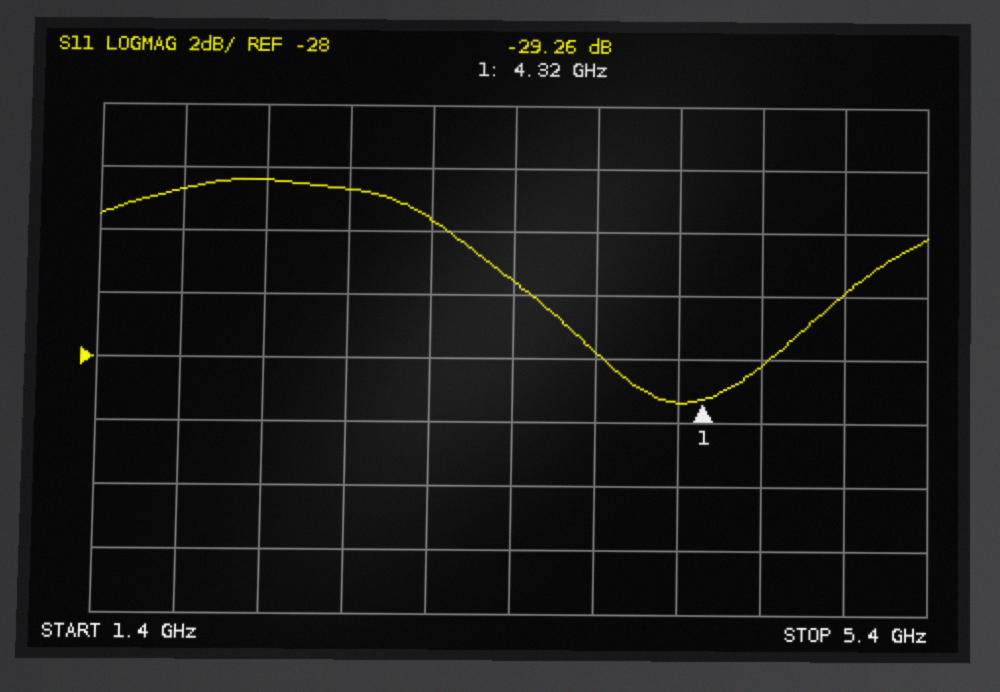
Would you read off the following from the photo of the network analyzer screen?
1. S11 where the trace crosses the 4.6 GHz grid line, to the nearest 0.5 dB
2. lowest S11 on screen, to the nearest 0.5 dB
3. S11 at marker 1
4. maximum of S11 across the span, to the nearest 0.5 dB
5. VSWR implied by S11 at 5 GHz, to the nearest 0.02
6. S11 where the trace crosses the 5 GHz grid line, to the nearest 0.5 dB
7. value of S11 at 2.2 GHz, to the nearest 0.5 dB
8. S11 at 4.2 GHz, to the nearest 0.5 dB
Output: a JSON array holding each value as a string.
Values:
["-28.0 dB", "-29.5 dB", "-29.26 dB", "-22.5 dB", "1.10", "-26.0 dB", "-22.5 dB", "-29.5 dB"]
